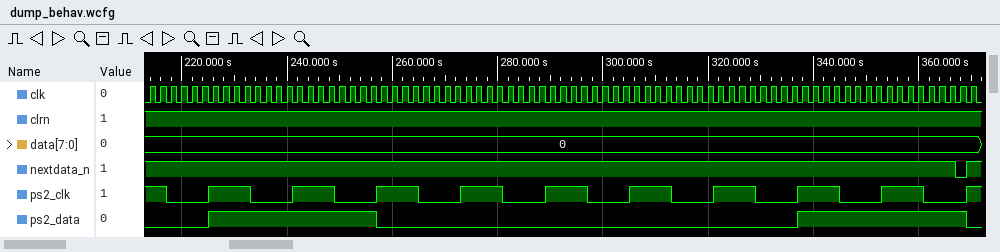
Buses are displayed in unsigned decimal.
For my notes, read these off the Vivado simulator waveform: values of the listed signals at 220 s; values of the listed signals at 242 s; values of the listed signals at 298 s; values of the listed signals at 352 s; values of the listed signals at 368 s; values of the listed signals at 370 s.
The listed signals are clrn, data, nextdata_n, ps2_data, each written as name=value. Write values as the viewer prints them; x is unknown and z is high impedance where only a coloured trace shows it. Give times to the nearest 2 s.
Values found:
clrn=1, data=0, nextdata_n=1, ps2_data=0
clrn=1, data=0, nextdata_n=1, ps2_data=1
clrn=1, data=0, nextdata_n=1, ps2_data=0
clrn=1, data=0, nextdata_n=1, ps2_data=1
clrn=1, data=0, nextdata_n=0, ps2_data=1
clrn=1, data=0, nextdata_n=1, ps2_data=0
